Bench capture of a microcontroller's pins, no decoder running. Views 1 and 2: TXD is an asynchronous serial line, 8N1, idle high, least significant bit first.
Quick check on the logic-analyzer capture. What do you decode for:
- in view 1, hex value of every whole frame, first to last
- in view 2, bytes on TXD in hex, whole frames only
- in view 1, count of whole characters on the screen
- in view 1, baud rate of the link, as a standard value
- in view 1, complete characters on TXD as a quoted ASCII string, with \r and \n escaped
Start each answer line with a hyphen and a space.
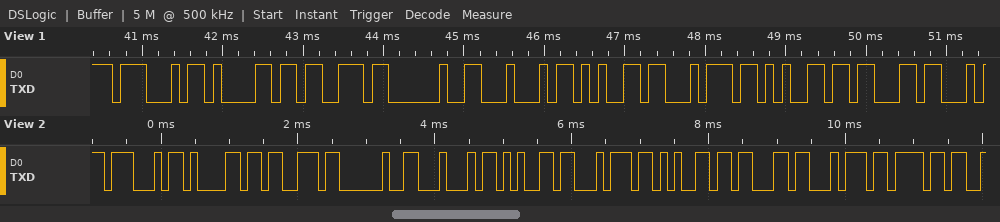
- 47 61 73 20 44 65 74 65 63
- 47 61 73 20 44 65 74 65 63 74 6F
- 9
- 9600 baud
- "Gas Detec"
